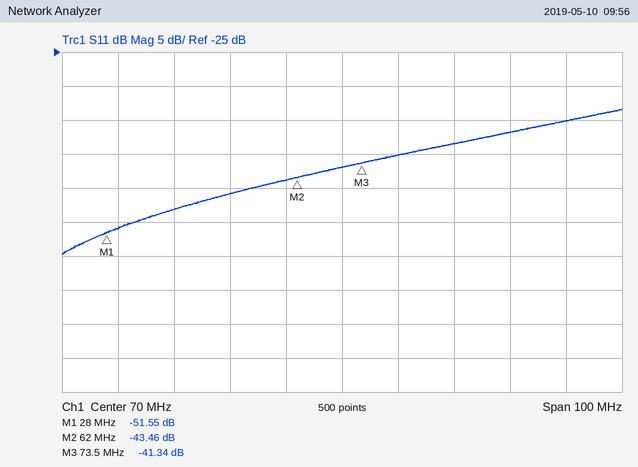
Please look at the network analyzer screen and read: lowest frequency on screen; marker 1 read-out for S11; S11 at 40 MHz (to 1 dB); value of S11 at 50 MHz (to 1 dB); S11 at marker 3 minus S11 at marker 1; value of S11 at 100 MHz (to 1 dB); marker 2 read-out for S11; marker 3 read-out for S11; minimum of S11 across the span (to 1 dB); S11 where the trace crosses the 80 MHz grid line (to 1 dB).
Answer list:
20 MHz
-51.55 dB
-48 dB
-46 dB
10.21 dB
-37 dB
-43.46 dB
-41.34 dB
-55 dB
-40 dB
